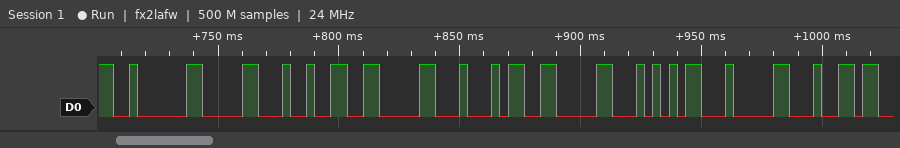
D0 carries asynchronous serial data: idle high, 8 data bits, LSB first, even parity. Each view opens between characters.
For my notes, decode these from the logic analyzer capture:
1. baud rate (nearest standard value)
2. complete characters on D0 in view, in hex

300 baud
02, 30, 32, 30, 34, 30, 35, 30
